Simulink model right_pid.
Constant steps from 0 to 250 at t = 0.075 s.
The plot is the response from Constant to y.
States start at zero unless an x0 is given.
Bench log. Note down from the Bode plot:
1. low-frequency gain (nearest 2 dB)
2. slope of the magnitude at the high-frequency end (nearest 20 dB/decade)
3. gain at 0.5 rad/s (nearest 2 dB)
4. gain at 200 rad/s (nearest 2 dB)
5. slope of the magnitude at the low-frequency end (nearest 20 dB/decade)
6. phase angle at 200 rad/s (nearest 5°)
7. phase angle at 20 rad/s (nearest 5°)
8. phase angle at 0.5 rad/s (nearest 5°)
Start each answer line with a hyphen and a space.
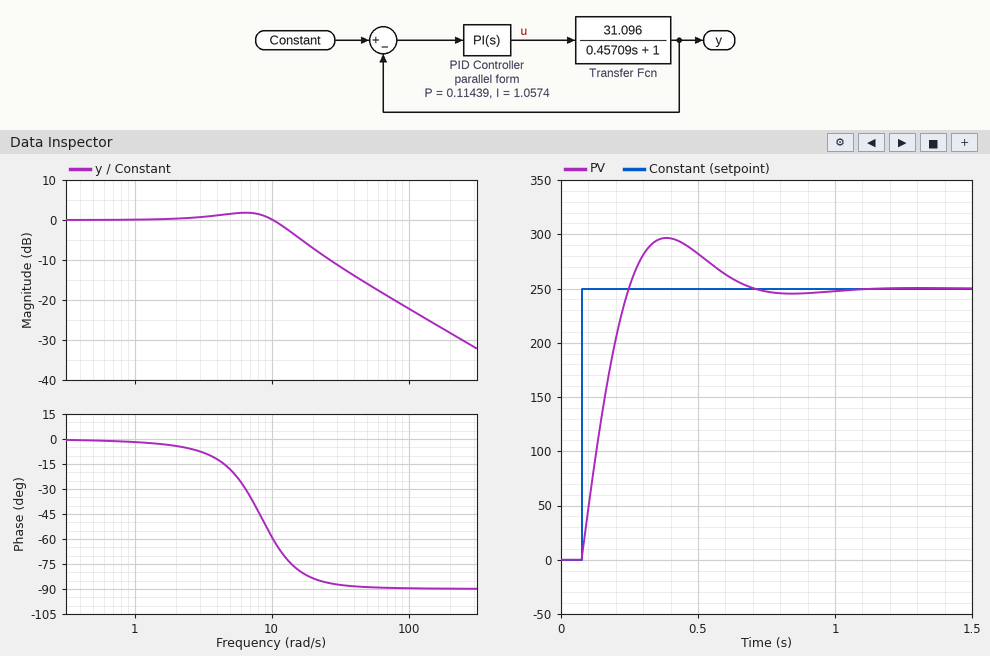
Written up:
- 0 dB
- -20 dB/decade
- 0 dB
- -28 dB
- 0 dB/decade
- -90°
- -85°
- 0°
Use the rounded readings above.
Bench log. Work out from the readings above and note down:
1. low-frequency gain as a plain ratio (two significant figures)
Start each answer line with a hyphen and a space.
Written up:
- 1.0
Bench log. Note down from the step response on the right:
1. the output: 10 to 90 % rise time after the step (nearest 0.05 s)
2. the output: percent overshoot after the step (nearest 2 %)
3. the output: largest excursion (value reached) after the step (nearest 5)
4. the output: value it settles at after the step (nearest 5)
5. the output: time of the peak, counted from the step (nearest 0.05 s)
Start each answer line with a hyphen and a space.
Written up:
- 0.15 s
- 18 %
- 295
- 250
- 0.30 s
